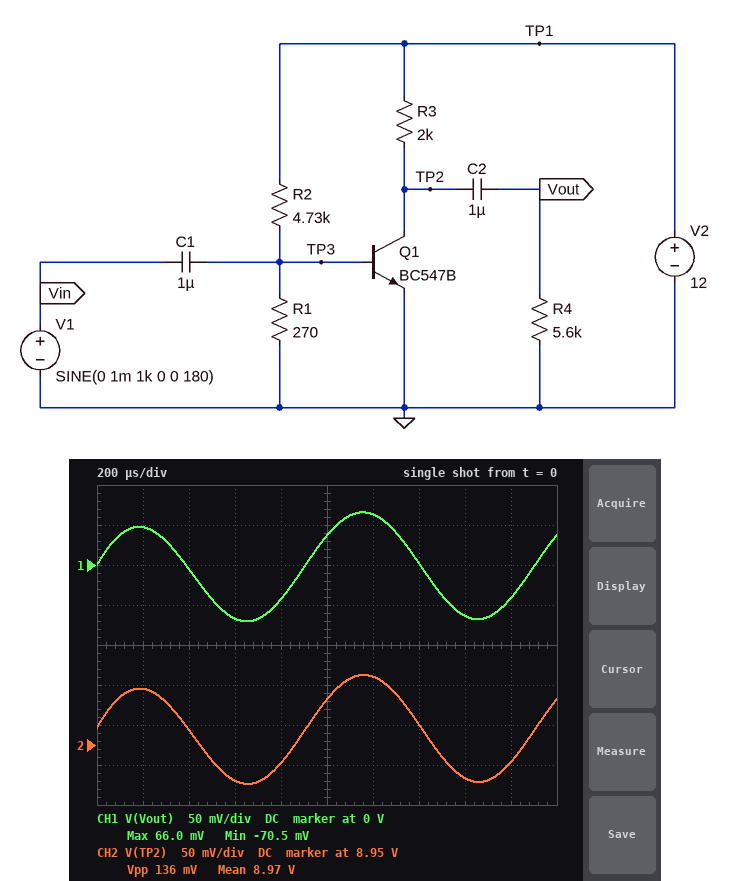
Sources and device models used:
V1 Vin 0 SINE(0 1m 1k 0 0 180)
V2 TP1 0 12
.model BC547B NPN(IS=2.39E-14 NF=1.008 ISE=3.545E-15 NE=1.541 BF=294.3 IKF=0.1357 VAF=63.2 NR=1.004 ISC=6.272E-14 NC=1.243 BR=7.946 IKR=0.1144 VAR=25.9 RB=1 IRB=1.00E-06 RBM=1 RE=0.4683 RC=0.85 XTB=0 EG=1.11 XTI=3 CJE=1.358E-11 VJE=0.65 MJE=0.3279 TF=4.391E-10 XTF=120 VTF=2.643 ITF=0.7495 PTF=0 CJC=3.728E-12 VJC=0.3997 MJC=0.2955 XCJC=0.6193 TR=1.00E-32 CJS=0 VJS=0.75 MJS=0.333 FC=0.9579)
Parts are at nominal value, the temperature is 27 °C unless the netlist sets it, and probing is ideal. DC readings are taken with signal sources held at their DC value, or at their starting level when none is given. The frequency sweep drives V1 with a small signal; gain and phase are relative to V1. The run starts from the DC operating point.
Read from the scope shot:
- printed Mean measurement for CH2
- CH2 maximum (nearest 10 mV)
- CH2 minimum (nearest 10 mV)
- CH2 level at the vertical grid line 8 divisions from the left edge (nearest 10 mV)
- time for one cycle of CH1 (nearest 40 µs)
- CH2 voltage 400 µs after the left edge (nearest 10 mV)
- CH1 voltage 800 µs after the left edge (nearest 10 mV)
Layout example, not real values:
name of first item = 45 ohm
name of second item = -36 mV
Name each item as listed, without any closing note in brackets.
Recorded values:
printed Mean measurement for CH2 = 8.97 V
CH2 maximum = 9.04 V
CH2 minimum = 8.90 V
CH2 level at the vertical grid line 8 divisions from the left edge = 8.91 V
time for one cycle of CH1 = 1.00 ms
CH2 voltage 400 µs after the left edge = 8.97 V
CH1 voltage 800 µs after the left edge = -40 mV
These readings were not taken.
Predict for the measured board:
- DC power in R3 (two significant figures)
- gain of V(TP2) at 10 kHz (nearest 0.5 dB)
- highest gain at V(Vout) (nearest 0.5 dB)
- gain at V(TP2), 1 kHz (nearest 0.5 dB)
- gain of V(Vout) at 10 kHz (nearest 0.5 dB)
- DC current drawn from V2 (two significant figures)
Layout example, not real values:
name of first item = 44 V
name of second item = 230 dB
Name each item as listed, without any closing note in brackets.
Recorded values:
DC power in R3 = 4.6 mW
gain of V(TP2) at 10 kHz = 38.0 dB
highest gain at V(Vout) = 38.0 dB
gain at V(TP2), 1 kHz = 36.5 dB
gain of V(Vout) at 10 kHz = 38.0 dB
DC current drawn from V2 = 3.9 mA
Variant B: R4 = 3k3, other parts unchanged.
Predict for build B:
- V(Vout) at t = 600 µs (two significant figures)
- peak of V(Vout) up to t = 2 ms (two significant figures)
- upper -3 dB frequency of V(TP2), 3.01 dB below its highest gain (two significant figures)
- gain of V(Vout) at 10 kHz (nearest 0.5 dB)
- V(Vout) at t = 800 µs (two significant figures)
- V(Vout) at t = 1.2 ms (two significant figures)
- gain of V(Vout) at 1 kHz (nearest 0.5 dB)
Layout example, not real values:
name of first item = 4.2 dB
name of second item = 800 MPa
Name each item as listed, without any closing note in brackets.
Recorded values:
V(Vout) at t = 600 µs = -57 mV
peak of V(Vout) up to t = 2 ms = 56 mV
upper -3 dB frequency of V(TP2), 3.01 dB below its highest gain = 84 MHz
gain of V(Vout) at 10 kHz = 36.5 dB
V(Vout) at t = 800 µs = -36 mV
V(Vout) at t = 1.2 ms = 54 mV
gain of V(Vout) at 1 kHz = 35.0 dB
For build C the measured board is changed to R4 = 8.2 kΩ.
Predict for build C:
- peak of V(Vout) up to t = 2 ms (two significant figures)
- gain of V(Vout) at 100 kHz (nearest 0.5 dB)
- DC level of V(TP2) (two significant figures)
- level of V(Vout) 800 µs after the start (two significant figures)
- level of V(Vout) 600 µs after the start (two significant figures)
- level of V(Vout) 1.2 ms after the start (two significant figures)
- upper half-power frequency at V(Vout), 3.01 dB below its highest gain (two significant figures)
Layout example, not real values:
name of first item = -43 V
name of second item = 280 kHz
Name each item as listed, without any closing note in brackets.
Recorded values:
peak of V(Vout) up to t = 2 ms = 72 mV
gain of V(Vout) at 100 kHz = 39.0 dB
DC level of V(TP2) = 9.0 V
level of V(Vout) 800 µs after the start = -47 mV
level of V(Vout) 600 µs after the start = -73 mV
level of V(Vout) 1.2 ms after the start = 69 mV
upper half-power frequency at V(Vout), 3.01 dB below its highest gain = 66 MHz
